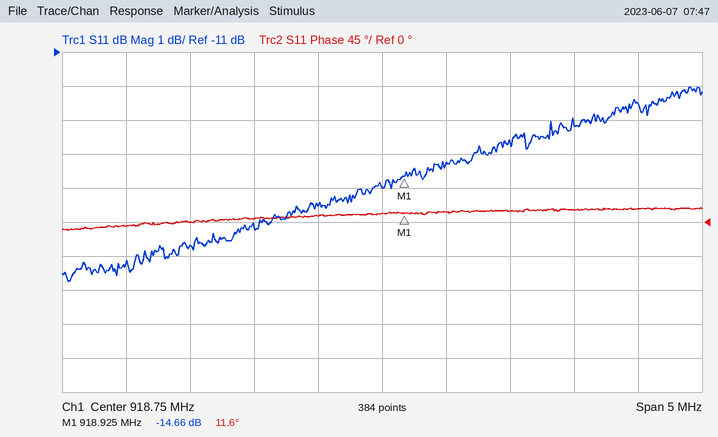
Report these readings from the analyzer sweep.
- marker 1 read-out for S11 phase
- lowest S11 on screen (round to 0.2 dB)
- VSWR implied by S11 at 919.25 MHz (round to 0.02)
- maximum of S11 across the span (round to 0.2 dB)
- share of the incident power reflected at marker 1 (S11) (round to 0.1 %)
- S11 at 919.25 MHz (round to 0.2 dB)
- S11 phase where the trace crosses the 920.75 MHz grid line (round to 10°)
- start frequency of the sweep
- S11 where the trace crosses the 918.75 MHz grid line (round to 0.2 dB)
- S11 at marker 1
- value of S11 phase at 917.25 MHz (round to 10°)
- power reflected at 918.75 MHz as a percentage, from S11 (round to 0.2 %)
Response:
11.6°
-17.8 dB
1.48
-12.0 dB
3.4 %
-14.2 dB
20°
916.25 MHz
-15.0 dB
-14.66 dB
0°
3.2 %
